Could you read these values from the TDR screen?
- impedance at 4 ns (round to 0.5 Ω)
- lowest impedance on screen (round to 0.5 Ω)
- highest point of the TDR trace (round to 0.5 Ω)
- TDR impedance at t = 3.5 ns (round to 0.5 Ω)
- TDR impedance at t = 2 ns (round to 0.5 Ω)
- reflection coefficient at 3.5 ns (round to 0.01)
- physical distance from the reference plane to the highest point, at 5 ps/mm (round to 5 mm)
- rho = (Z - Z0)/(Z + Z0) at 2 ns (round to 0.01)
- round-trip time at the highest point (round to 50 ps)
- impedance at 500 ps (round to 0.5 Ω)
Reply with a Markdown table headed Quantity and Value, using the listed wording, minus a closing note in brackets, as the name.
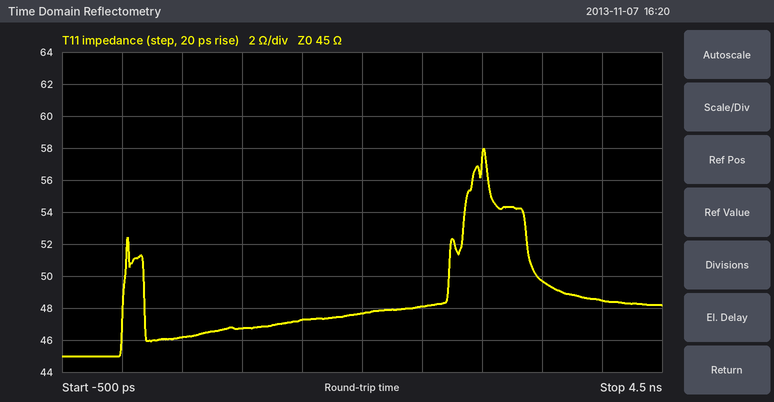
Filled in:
| Quantity | Value |
|---|---|
| impedance at 4 ns | 48.5 Ω |
| lowest impedance on screen | 45.0 Ω |
| highest point of the TDR trace | 58.0 Ω |
| TDR impedance at t = 3.5 ns | 49.5 Ω |
| TDR impedance at t = 2 ns | 47.5 Ω |
| reflection coefficient at 3.5 ns | +0.05 |
| physical distance from the reference plane to the highest point, at 5 ps/mm | 300 mm |
| rho = (Z - Z0)/(Z + Z0) at 2 ns | +0.03 |
| round-trip time at the highest point | 3.00 ns |
| impedance at 500 ps | 46.0 Ω |
